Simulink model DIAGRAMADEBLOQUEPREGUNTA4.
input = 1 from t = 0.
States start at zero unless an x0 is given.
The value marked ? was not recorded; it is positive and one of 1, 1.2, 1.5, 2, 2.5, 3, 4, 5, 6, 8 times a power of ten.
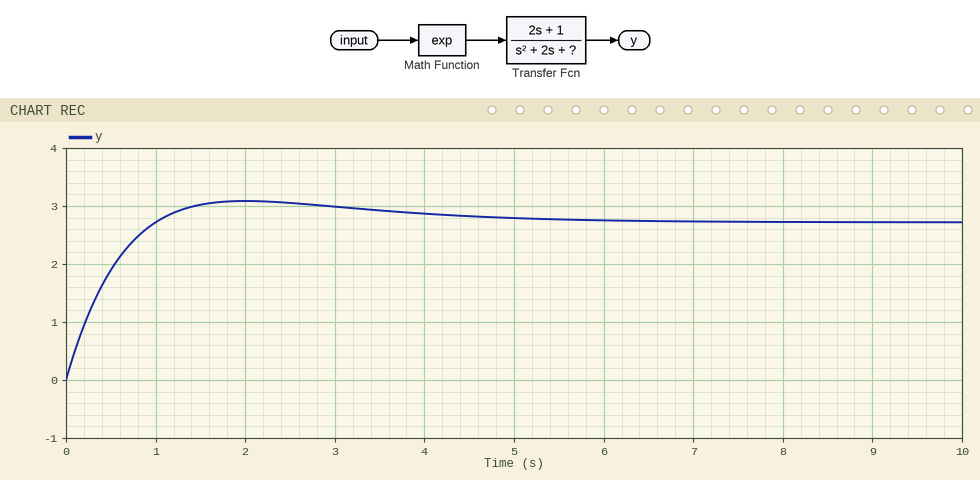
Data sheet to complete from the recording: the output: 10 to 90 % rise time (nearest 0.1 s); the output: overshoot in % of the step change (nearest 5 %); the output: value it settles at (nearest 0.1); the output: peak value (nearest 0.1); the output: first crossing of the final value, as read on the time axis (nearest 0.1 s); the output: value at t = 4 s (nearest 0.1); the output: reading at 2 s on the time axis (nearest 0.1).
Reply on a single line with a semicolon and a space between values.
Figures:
0.7 s; 15 %; 2.7; 3.1; 1.0 s; 2.9; 3.1
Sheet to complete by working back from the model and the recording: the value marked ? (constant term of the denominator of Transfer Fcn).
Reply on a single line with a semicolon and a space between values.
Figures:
1
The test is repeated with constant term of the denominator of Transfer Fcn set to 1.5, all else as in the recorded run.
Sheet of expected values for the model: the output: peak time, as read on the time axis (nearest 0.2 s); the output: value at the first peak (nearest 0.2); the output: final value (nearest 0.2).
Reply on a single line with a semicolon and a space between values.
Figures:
1.4 s; 2.6; 1.8
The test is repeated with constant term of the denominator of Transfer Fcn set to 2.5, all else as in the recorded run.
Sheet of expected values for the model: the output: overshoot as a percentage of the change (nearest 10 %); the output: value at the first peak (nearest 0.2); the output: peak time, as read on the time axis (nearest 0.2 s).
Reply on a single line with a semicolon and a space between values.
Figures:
100 %; 2.2; 1.0 s
